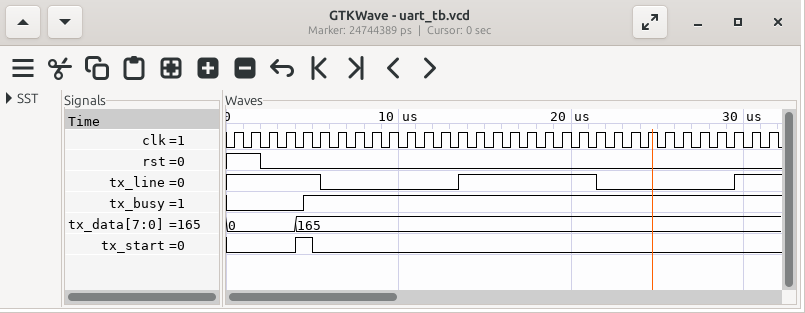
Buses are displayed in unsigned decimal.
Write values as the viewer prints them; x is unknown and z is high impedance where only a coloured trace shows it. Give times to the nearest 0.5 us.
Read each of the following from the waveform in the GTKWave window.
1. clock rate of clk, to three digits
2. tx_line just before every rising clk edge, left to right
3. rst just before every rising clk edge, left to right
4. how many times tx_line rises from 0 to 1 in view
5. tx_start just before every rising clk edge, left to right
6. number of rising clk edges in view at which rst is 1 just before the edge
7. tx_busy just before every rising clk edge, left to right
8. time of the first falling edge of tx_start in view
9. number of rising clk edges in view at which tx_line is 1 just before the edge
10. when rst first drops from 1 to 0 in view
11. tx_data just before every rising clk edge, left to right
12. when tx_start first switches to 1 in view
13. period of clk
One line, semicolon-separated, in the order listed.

1.00 MHz; 1 1 1 1 1 1 0 0 0 0 0 0 0 0 1 1 1 1 1 1 1 1 0 0 0 0 0 0 0 0 1 1; 1 1 0 0 0 0 0 0 0 0 0 0 0 0 0 0 0 0 0 0 0 0 0 0 0 0 0 0 0 0 0 0; 2; 0 0 0 0 1 0 0 0 0 0 0 0 0 0 0 0 0 0 0 0 0 0 0 0 0 0 0 0 0 0 0 0; 2; 0 0 0 0 0 1 1 1 1 1 1 1 1 1 1 1 1 1 1 1 1 1 1 1 1 1 1 1 1 1 1 1; 5 us; 16; 2 us; 0, 0, 0, 0, 165, 165, 165, 165, 165, 165, 165, 165, 165, 165, 165, 165, 165, 165, 165, 165, 165, 165, 165, 165, 165, 165, 165, 165, 165, 165, 165, 165; 4 us; 1 us
